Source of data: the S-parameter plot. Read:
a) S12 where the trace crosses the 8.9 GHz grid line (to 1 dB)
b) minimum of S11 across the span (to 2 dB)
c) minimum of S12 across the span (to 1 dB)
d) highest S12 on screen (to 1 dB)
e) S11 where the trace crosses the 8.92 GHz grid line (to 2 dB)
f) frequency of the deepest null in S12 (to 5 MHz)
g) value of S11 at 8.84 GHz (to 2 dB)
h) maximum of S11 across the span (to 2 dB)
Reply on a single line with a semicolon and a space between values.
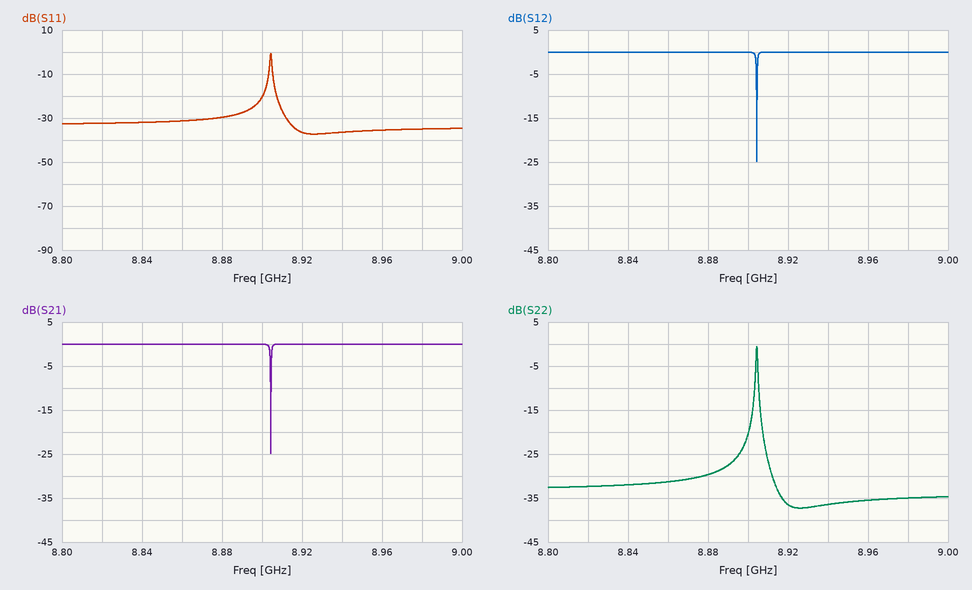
0 dB; -38 dB; -25 dB; 0 dB; -36 dB; 8.905 GHz; -32 dB; 0 dB
